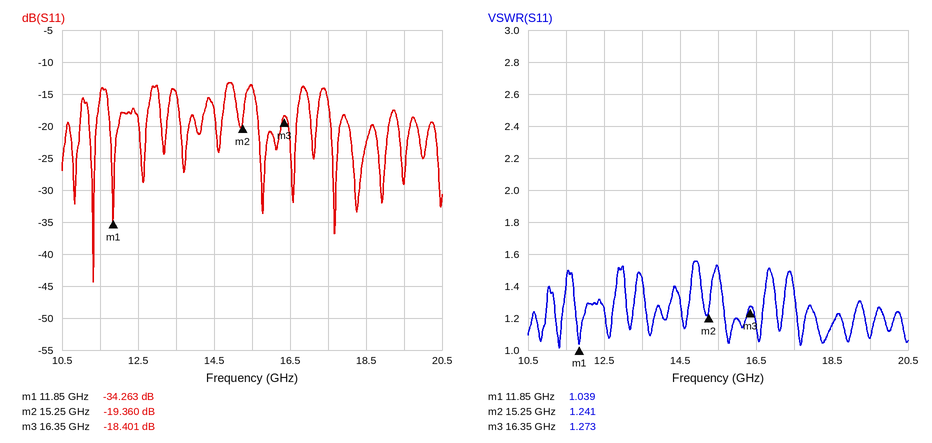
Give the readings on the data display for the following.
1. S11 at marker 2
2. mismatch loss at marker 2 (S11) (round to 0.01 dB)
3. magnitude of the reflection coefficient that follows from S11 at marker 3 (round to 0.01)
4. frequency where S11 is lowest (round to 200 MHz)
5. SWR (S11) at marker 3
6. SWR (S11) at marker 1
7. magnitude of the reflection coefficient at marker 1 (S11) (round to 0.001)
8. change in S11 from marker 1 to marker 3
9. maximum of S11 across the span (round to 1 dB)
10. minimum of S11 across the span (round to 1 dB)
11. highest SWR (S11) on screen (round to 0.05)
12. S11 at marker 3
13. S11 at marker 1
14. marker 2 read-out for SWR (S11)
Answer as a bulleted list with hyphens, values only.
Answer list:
- -19.360 dB
- 0.05 dB
- 0.12
- 11.4 GHz
- 1.273
- 1.039
- 0.019
- 15.862 dB
- -13 dB
- -44 dB
- 1.55
- -18.401 dB
- -34.263 dB
- 1.241
